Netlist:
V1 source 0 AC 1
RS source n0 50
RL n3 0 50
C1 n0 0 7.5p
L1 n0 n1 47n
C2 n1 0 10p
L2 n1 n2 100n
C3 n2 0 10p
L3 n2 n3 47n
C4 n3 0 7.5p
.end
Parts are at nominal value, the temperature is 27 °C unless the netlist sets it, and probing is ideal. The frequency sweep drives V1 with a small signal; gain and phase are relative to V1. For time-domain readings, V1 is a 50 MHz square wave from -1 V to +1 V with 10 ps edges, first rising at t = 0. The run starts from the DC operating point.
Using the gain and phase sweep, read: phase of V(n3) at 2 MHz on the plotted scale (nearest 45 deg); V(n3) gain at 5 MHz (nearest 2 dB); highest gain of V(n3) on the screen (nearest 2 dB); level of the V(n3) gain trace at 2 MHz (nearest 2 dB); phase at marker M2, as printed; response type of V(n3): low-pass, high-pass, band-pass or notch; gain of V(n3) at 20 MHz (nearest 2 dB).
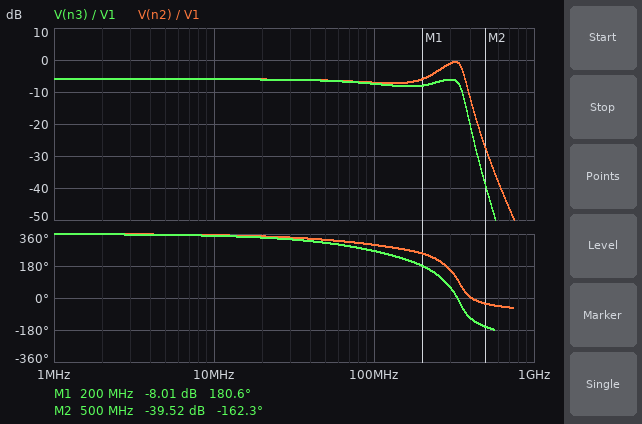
360 deg
-6 dB
-6 dB
-6 dB
-162.3 deg
low-pass
-6 dB
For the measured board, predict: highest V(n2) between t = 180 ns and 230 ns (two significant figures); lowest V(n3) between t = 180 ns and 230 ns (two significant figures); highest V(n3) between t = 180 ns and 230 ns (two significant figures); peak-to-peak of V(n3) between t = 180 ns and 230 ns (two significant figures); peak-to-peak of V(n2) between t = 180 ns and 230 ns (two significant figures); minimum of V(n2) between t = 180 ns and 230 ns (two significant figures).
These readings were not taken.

700 mV
-570 mV
570 mV
1.1 V
1.4 V
-700 mV
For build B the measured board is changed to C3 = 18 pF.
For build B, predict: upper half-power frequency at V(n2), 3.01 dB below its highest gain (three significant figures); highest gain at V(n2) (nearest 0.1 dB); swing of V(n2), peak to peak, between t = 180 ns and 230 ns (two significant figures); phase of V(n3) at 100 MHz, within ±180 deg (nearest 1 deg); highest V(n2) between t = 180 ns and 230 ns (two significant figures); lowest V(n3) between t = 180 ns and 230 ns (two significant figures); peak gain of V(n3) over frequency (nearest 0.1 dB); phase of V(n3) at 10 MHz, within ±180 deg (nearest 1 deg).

328 MHz
-5.6 dB
1.3 V
-106 deg
630 mV
-550 mV
-6.0 dB
-11 deg
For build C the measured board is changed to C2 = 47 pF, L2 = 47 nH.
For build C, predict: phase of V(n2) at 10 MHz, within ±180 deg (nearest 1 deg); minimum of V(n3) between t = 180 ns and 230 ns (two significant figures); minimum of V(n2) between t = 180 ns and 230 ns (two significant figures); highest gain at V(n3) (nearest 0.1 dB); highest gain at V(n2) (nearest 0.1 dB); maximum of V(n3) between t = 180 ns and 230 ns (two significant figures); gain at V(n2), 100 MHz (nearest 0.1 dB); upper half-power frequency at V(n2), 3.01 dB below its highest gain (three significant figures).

-8 deg
-560 mV
-570 mV
-6.0 dB
-6.0 dB
560 mV
-6.5 dB
164 MHz
